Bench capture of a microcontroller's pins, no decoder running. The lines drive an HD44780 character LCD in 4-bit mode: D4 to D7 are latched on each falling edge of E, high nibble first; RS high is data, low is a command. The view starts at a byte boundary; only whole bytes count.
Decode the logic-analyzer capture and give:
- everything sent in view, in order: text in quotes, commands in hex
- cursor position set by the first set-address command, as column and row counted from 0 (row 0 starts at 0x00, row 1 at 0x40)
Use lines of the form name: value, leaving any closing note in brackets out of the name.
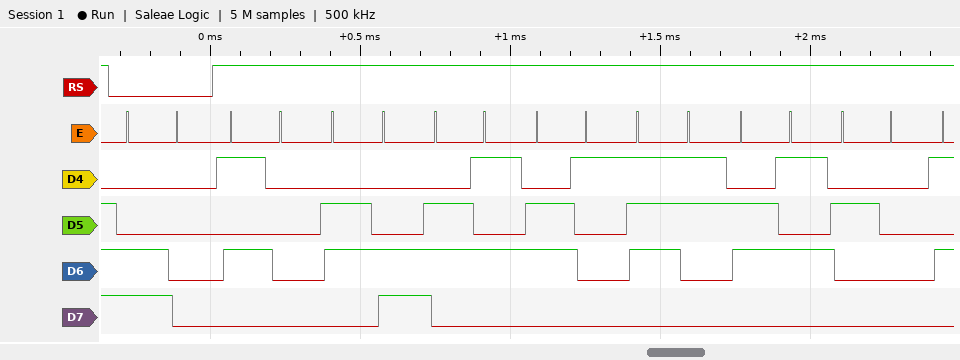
everything sent in view, in order: text in quotes, commands in hex: 0xC0 "Please "
cursor position set by the first set-address command, as column and row counted from 0: column 0, row 1
